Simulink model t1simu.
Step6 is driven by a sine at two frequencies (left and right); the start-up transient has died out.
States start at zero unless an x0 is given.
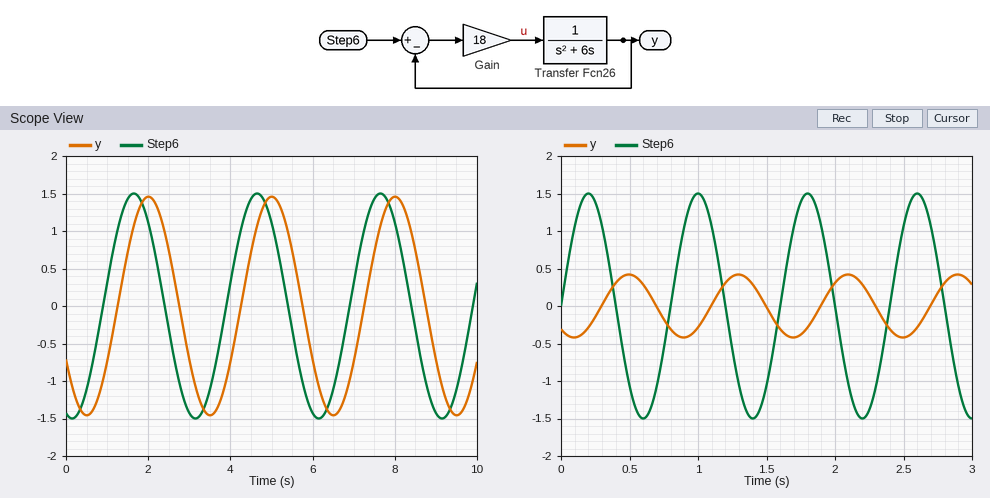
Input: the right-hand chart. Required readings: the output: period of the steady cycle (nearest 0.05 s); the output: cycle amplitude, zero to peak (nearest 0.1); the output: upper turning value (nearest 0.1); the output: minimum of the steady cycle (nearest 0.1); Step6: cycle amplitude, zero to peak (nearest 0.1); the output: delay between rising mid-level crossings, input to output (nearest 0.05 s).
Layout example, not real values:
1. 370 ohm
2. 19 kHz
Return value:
1. 0.80 s
2. 0.4
3. 0.4
4. -0.4
5. 1.5
6. 0.30 s
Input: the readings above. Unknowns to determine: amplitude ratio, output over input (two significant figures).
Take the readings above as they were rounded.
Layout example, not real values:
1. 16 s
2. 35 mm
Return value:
1. 0.27
